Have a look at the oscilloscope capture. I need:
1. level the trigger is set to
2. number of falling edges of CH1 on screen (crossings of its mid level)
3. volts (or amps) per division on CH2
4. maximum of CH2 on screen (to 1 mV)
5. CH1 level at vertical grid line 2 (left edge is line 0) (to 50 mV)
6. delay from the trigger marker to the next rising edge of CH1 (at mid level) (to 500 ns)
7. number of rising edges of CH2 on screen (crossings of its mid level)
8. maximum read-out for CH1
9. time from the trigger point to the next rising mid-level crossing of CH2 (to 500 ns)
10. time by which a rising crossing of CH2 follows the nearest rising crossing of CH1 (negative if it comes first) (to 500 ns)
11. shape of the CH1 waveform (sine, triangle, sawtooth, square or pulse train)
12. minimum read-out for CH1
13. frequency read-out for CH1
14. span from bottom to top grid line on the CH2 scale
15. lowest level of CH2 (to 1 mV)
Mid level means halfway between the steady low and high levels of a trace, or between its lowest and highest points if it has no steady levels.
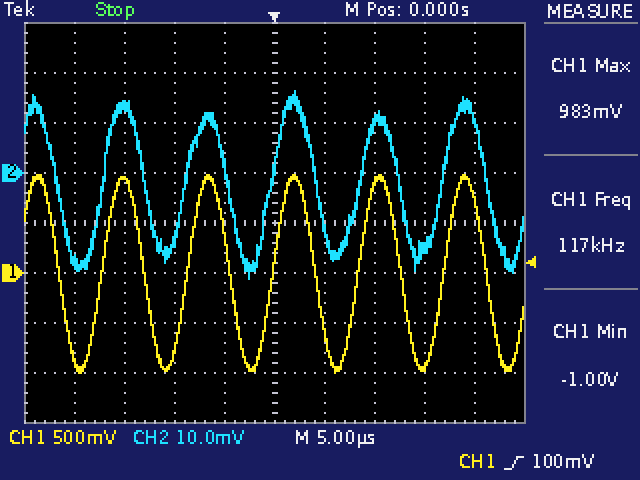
100 mV
6
10 mV
16 mV
950 mV
8.5 µs
5
983 mV
8.5 µs
0.0 µs
sine
-1.00 V
117 kHz
80 mV
-21 mV
